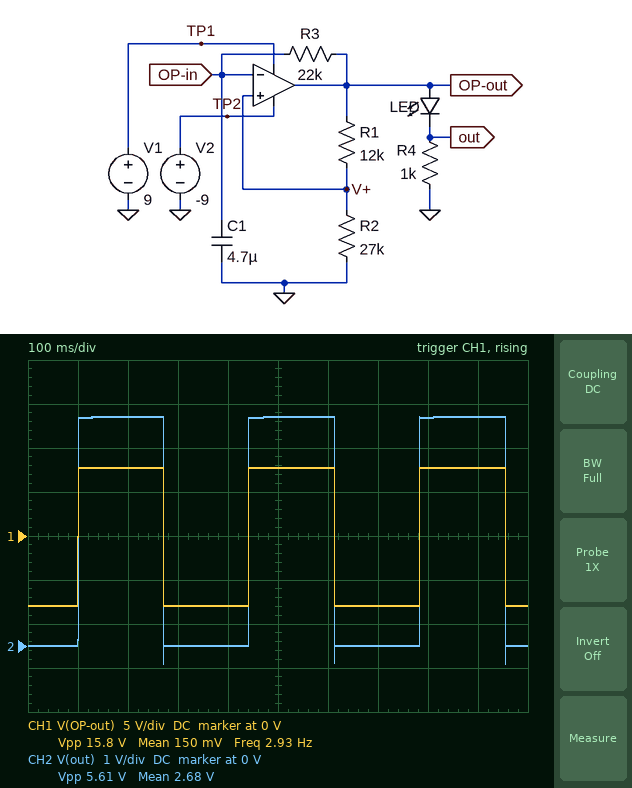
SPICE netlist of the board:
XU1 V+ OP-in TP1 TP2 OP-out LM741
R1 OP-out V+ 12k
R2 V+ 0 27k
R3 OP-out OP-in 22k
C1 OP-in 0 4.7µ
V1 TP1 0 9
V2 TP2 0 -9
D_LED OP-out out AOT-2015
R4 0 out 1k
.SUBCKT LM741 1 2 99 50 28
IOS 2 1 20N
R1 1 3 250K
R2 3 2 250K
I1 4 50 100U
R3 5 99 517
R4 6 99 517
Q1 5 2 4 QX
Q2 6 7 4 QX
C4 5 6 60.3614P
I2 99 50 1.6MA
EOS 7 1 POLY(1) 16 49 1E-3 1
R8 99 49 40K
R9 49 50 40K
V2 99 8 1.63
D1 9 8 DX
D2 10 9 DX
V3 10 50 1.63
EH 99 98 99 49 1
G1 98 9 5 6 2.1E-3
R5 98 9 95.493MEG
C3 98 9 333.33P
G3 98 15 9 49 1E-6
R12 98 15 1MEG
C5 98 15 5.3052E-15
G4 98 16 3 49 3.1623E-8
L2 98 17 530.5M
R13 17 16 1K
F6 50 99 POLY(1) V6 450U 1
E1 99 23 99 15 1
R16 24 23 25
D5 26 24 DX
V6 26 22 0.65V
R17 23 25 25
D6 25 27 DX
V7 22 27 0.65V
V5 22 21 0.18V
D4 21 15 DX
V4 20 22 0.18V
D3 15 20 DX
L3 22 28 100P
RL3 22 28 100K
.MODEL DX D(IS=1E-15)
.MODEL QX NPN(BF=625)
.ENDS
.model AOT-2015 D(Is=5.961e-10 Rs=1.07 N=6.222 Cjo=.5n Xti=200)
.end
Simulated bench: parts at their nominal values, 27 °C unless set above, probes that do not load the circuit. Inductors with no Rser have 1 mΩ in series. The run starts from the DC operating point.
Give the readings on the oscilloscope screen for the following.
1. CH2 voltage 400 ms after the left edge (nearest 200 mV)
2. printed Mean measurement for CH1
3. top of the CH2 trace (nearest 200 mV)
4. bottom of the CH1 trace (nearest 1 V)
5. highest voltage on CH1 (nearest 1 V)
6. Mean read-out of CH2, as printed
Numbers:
0 V
150 mV
5.2 V
-8 V
8 V
2.68 V
